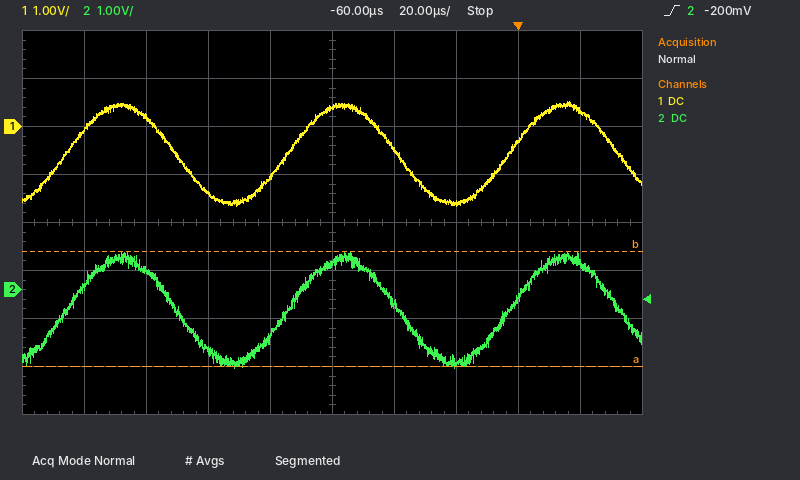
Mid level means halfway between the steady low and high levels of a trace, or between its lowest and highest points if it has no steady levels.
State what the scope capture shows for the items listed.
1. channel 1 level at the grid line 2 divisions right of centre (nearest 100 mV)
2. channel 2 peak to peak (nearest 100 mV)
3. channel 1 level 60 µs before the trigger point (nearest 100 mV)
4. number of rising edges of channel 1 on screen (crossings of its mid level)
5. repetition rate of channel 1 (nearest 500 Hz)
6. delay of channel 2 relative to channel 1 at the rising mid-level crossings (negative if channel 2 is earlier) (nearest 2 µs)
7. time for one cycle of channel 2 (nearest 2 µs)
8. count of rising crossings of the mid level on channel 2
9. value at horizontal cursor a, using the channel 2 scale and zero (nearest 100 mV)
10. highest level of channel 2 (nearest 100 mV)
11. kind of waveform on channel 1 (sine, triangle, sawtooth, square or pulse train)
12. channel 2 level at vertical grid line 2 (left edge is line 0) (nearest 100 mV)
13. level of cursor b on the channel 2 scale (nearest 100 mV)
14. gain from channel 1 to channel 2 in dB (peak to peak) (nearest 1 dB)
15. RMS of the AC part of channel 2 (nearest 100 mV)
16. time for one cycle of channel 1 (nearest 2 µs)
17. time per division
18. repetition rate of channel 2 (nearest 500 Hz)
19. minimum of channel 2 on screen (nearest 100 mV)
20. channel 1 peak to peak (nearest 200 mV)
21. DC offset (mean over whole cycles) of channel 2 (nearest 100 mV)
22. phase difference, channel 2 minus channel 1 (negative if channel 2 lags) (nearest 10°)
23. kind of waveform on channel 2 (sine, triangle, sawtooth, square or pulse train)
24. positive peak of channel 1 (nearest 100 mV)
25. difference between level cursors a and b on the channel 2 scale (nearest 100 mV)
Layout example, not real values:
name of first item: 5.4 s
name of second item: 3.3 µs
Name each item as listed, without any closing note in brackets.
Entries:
channel 1 level at the grid line 2 divisions right of centre: -1.6 V
channel 2 peak to peak: 2.4 V
channel 1 level 60 µs before the trigger point: 400 mV
number of rising edges of channel 1 on screen: 3
repetition rate of channel 1: 14.0 kHz
delay of channel 2 relative to channel 1 at the rising mid-level crossings (negative if channel 2 is earlier): 0 µs
time for one cycle of channel 2: 72 µs
count of rising crossings of the mid level on channel 2: 3
value at horizontal cursor a, using the channel 2 scale and zero: -1.6 V
highest level of channel 2: 800 mV
kind of waveform on channel 1: sine
channel 2 level at vertical grid line 2 (left edge is line 0): 400 mV
level of cursor b on the channel 2 scale: 800 mV
gain from channel 1 to channel 2 in dB (peak to peak): 1 dB
RMS of the AC part of channel 2: 800 mV
time for one cycle of channel 1: 72 µs
time per division: 20 µs
repetition rate of channel 2: 14.0 kHz
minimum of channel 2 on screen: -1.6 V
channel 1 peak to peak: 2.2 V
DC offset (mean over whole cycles) of channel 2: -400 mV
phase difference, channel 2 minus channel 1 (negative if channel 2 lags): 0°
kind of waveform on channel 2: sine
positive peak of channel 1: 500 mV
difference between level cursors a and b on the channel 2 scale: 2.4 V
